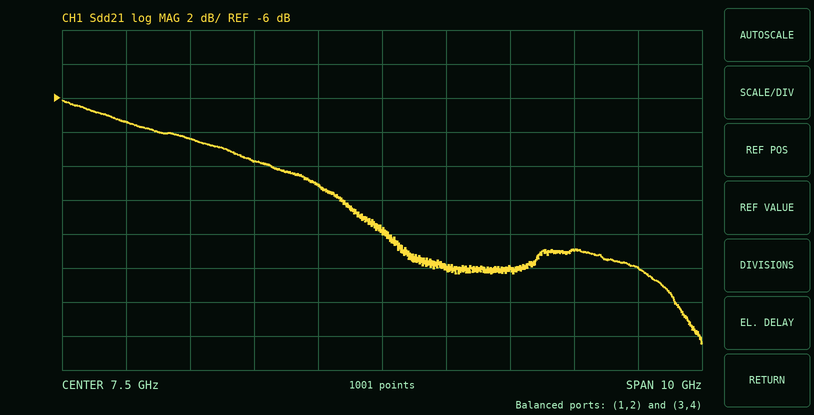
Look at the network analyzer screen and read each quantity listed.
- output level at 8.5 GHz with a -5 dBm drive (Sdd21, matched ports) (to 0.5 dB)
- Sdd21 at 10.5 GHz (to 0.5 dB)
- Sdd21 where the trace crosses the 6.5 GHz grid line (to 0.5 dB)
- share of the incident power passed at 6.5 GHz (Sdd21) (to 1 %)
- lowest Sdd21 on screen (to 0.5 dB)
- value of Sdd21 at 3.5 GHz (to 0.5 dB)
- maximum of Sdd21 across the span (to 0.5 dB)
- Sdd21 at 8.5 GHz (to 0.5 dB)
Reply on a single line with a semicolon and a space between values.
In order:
-21.0 dBm; -15.0 dB; -11.0 dB; 8 %; -20.5 dB; -7.5 dB; -6.0 dB; -16.0 dB
